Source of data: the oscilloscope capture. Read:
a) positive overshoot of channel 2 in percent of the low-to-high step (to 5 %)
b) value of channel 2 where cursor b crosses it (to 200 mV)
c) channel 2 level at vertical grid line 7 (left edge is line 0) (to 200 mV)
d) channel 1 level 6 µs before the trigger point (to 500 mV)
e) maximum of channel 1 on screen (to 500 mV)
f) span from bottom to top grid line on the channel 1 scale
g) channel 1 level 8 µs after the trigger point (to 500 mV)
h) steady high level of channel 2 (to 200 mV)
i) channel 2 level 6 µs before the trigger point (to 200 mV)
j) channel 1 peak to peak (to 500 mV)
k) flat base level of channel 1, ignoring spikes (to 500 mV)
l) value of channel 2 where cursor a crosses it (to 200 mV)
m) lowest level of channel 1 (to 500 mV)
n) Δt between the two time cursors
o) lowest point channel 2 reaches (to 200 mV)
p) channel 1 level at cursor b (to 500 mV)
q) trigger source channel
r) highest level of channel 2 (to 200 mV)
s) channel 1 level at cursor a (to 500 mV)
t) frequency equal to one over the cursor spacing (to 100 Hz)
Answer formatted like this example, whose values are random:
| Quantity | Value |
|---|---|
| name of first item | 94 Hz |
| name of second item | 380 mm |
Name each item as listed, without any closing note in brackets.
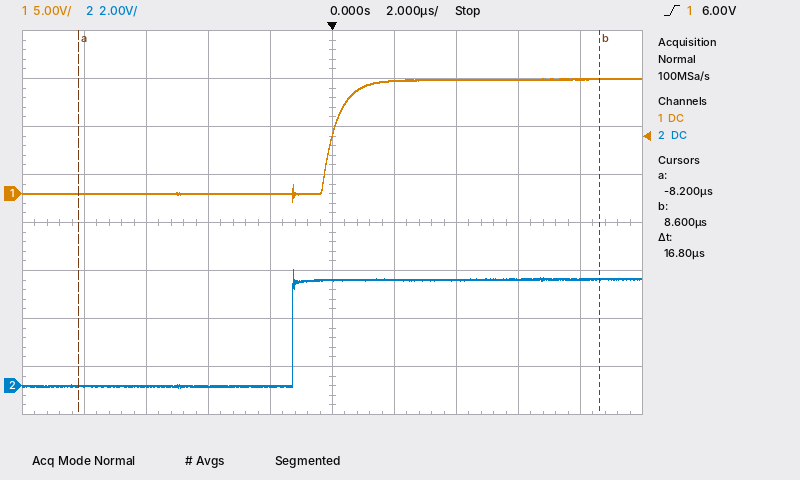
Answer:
| Quantity | Value |
|---|---|
| positive overshoot of channel 2 in percent of the low-to-high step | 10 % |
| value of channel 2 where cursor b crosses it | 4.4 V |
| channel 2 level at vertical grid line 7 (left edge is line 0) | 4.4 V |
| channel 1 level 6 µs before the trigger point | 0.0 V |
| maximum of channel 1 on screen | 12.0 V |
| span from bottom to top grid line on the channel 1 scale | 40 V |
| channel 1 level 8 µs after the trigger point | 12.0 V |
| steady high level of channel 2 | 4.4 V |
| channel 2 level 6 µs before the trigger point | 0.0 V |
| channel 1 peak to peak | 13.0 V |
| flat base level of channel 1, ignoring spikes | 0.0 V |
| value of channel 2 where cursor a crosses it | 0.0 V |
| lowest level of channel 1 | -1.0 V |
| Δt between the two time cursors | 16.8 µs |
| lowest point channel 2 reaches | 0.0 V |
| channel 1 level at cursor b | 12.0 V |
| trigger source channel | channel 1 |
| highest level of channel 2 | 4.8 V |
| channel 1 level at cursor a | 0.0 V |
| frequency equal to one over the cursor spacing | 59.5 kHz |
